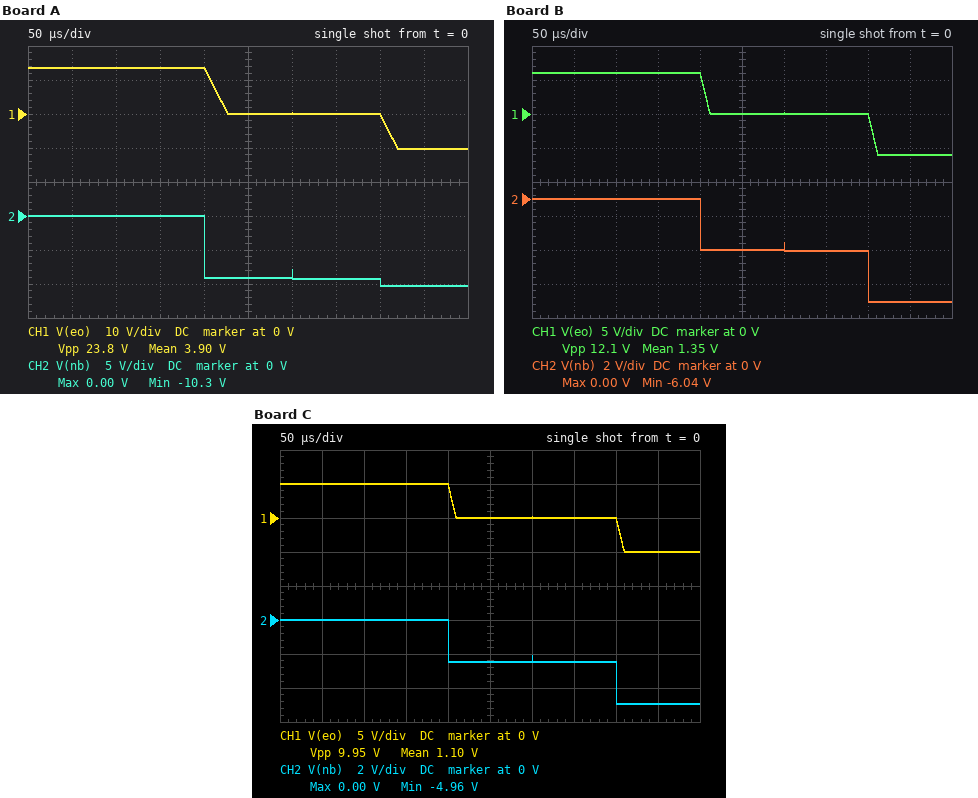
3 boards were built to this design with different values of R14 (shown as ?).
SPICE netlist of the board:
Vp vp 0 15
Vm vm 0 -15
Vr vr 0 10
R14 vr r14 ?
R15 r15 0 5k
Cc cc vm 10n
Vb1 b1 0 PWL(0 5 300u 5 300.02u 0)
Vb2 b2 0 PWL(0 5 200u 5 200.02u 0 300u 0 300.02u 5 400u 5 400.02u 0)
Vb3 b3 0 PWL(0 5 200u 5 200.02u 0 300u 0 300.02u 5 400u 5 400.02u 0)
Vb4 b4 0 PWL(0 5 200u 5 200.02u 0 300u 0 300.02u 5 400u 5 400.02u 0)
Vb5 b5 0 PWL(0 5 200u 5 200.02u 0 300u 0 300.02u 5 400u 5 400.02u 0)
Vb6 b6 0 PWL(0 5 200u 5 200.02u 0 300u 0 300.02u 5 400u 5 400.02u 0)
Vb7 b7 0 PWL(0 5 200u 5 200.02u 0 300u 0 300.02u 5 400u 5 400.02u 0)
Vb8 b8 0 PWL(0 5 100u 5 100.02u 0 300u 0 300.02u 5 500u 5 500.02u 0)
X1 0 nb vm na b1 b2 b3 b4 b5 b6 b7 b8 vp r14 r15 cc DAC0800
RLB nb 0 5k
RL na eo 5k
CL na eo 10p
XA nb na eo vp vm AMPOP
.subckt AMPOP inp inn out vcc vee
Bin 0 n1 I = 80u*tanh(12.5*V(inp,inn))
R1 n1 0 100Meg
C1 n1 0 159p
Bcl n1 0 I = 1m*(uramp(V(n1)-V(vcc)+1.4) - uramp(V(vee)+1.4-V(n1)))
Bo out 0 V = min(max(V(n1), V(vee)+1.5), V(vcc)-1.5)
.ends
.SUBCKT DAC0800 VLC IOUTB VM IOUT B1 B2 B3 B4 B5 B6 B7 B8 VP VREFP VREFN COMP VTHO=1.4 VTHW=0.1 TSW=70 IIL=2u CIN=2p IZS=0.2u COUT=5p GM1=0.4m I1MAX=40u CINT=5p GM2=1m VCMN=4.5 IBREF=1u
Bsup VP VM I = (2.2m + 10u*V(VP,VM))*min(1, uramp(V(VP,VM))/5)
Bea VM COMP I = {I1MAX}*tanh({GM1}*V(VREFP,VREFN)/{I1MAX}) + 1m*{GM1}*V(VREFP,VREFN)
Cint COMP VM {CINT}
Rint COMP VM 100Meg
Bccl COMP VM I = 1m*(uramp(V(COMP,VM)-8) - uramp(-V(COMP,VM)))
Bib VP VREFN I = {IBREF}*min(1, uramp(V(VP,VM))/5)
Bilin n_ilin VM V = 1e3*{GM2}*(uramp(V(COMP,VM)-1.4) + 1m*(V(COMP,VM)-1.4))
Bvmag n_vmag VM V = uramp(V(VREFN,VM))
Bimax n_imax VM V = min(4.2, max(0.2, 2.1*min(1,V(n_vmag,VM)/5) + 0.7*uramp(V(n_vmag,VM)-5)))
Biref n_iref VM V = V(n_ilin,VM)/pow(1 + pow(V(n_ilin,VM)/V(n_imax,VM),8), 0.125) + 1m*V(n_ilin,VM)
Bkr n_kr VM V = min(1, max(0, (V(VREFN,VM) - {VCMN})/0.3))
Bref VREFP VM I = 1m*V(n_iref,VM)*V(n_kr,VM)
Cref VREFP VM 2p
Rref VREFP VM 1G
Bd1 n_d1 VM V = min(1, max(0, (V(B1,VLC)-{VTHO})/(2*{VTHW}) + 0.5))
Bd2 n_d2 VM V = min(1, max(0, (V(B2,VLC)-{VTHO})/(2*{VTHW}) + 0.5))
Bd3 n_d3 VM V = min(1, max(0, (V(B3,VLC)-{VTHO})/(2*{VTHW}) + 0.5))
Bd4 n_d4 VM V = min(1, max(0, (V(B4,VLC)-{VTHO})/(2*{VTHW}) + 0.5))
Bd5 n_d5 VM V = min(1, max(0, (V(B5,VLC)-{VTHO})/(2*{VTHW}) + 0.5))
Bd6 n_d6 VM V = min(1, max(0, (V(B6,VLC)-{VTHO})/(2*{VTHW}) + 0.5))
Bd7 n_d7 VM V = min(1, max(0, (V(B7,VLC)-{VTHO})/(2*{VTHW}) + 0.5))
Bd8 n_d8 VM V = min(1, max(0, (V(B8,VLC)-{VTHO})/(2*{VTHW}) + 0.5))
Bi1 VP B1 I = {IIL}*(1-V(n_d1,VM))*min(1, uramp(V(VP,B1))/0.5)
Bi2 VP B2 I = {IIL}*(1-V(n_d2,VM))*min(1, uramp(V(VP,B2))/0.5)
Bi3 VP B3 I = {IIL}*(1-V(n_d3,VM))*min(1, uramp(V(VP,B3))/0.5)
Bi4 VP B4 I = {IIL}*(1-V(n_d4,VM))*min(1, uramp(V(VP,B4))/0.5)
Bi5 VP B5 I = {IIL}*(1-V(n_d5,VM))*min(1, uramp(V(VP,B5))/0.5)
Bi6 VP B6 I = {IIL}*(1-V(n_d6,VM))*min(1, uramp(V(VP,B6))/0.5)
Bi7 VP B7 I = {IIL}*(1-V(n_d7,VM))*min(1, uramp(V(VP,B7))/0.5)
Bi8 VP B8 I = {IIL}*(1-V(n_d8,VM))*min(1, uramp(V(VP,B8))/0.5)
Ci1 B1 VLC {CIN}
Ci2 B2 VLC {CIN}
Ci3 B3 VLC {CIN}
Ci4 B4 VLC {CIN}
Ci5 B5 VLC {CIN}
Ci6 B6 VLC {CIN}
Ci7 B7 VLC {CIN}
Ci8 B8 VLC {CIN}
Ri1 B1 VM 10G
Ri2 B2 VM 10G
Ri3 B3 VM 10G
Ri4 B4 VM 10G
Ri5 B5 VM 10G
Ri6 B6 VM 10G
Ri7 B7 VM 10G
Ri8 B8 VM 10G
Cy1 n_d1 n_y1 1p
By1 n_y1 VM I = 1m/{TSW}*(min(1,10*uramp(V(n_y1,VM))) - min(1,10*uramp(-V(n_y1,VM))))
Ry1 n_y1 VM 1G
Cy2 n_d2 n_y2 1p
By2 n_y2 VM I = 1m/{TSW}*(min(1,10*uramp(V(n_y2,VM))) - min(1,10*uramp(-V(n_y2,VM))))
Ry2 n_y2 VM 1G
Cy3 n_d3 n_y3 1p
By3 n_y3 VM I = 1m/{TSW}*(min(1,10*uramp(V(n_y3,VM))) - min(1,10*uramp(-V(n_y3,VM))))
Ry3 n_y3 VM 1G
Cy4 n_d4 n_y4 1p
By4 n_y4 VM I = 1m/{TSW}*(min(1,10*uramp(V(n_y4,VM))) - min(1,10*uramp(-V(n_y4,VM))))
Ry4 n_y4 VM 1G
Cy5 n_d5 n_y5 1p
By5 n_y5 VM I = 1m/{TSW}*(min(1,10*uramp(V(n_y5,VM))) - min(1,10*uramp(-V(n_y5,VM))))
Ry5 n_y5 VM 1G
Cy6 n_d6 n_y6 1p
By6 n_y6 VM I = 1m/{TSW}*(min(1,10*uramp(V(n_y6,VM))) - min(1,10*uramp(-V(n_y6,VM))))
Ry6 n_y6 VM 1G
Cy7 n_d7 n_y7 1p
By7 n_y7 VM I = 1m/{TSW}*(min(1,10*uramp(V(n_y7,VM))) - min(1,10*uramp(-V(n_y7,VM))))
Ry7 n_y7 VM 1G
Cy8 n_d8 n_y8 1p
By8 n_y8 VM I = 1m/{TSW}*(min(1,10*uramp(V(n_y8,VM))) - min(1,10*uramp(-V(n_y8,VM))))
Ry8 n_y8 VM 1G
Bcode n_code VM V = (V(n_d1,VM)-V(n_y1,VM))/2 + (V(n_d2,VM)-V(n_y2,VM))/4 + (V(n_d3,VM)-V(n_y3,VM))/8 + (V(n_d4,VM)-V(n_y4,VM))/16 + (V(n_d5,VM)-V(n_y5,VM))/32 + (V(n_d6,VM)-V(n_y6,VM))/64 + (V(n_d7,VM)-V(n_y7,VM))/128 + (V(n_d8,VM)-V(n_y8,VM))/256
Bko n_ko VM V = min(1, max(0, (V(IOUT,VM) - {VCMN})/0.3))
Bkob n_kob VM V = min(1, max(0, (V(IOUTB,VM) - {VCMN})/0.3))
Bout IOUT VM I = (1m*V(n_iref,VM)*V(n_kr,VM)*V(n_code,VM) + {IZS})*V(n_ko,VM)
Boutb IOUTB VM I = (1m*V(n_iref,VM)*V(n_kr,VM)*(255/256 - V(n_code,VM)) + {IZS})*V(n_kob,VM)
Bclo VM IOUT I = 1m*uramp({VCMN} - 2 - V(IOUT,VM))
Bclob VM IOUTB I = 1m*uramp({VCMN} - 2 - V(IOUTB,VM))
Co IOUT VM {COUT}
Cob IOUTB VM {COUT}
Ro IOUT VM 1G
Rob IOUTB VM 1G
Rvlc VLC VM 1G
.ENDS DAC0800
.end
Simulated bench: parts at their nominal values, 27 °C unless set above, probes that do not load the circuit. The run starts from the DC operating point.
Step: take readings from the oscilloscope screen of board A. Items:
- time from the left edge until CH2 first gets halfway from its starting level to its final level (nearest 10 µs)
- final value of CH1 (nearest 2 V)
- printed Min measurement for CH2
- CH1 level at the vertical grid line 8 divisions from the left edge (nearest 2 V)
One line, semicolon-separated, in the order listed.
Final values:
200 µs; -10 V; -10.3 V; 0 V
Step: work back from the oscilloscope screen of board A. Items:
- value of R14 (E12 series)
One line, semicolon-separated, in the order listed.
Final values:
2.7 kΩ
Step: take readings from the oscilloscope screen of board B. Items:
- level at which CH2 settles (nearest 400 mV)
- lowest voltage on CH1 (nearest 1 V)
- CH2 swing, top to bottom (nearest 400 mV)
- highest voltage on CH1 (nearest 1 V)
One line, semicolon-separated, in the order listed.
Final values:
-6.0 V; -6 V; 6.0 V; 6 V
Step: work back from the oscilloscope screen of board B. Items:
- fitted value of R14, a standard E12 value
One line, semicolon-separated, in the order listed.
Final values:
8.2 kΩ
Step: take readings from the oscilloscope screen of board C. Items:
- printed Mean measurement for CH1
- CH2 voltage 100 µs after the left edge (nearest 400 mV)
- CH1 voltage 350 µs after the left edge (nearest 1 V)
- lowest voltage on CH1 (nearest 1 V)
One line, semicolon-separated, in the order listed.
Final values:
1.10 V; 0 V; 0 V; -5 V
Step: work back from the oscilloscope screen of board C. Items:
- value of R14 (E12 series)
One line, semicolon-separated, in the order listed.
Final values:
10 kΩ
